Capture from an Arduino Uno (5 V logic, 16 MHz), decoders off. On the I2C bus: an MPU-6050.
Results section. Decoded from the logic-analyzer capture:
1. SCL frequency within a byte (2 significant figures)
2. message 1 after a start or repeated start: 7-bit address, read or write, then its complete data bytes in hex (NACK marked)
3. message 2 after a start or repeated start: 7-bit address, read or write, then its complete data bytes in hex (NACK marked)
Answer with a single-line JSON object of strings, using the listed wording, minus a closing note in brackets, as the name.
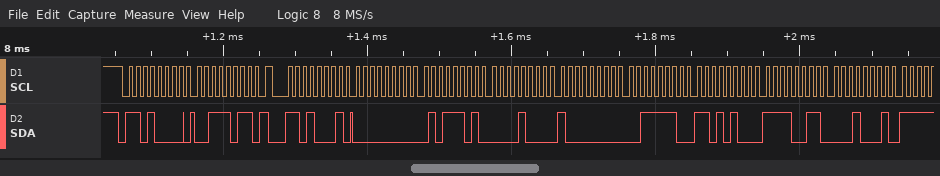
{"SCL frequency within a byte": "100 kHz", "message 1 after a start or repeated start: 7-bit address, read or write, then its complete data bytes in hex": "0x68 write: 3B", "message 2 after a start or repeated start: 7-bit address, read or write, then its complete data bytes in hex": "0x68 read: 00 5D 08 80 3E D4 F3 11"}
